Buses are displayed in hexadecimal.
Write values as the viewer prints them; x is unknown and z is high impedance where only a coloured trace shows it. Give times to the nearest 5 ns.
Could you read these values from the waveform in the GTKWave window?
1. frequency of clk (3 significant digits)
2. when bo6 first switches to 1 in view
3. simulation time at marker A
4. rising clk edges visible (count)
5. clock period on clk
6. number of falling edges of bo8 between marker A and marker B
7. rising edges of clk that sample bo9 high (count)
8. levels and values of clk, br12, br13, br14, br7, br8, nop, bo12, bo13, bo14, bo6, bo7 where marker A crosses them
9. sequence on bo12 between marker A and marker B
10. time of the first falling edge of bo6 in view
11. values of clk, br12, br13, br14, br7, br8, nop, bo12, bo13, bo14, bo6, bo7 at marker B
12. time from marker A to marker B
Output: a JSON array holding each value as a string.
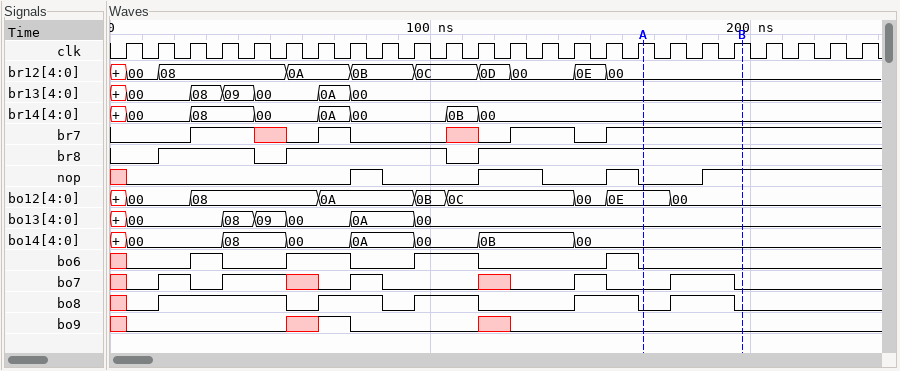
["100 MHz", "25 ns", "165 ns", "24", "10 ns", "1", "1", "clk=1, br12=00, br13=00, br14=00, br7=1, br8=1, nop=0, bo12=0E, bo13=00, bo14=00, bo6=0, bo7=0", "0E, 00", "35 ns", "clk=1, br12=00, br13=00, br14=00, br7=1, br8=1, nop=1, bo12=00, bo13=00, bo14=00, bo6=0, bo7=0", "30 ns"]
